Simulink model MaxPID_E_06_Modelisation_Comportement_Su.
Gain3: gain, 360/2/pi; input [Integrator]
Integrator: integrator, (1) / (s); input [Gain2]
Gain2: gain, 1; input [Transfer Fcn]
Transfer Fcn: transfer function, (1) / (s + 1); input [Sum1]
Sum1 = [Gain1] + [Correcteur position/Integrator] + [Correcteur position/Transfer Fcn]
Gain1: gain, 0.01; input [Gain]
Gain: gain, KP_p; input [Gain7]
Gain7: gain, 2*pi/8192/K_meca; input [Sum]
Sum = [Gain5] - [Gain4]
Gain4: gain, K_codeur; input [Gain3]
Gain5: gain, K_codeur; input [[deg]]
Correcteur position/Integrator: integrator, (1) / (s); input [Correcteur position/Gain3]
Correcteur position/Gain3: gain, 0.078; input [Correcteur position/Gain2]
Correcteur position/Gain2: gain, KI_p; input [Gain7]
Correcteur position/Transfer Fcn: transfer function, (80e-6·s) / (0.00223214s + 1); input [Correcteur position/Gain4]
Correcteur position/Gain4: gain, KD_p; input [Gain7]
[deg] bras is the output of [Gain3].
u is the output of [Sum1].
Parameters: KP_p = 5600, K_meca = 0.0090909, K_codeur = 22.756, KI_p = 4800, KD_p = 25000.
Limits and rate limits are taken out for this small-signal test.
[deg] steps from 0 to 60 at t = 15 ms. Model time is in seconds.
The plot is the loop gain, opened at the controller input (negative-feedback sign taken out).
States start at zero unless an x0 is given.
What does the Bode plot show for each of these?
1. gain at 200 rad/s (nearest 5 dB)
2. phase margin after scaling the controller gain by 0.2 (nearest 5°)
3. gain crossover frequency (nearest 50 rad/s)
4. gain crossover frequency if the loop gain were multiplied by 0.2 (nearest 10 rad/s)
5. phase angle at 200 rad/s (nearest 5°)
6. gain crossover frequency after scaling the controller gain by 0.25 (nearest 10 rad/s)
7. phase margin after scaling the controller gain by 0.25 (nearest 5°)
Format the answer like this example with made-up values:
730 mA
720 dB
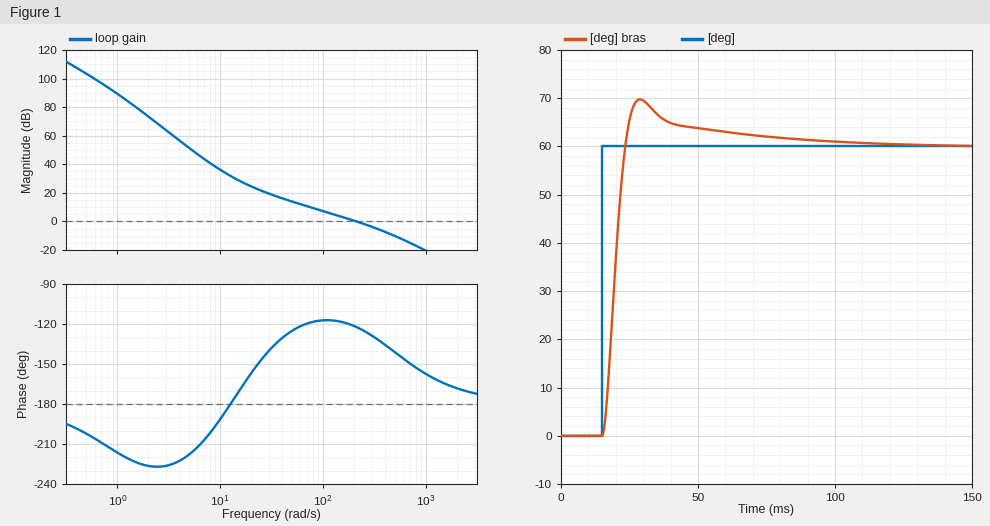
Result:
0 dB
55°
200 rad/s
50 rad/s
-120°
60 rad/s
60°
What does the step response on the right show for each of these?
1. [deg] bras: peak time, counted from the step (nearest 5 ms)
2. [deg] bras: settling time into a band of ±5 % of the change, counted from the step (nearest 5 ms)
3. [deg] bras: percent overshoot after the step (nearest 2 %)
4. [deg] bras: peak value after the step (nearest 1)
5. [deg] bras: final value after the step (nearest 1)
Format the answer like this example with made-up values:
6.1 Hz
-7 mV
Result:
15 ms
45 ms
16 %
70
60
